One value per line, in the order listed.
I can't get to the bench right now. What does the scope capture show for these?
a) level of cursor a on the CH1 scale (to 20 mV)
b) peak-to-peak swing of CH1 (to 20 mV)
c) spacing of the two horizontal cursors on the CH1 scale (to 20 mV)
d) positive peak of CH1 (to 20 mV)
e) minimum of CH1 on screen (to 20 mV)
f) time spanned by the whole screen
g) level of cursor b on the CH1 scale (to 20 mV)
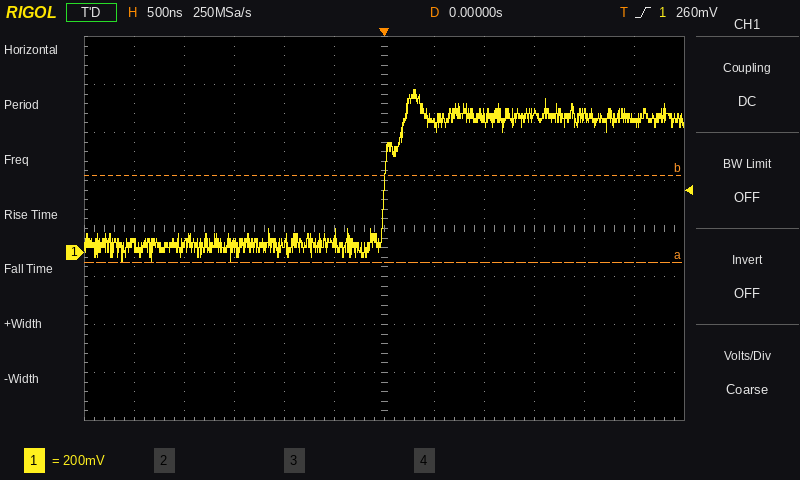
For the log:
-40 mV
720 mV
360 mV
680 mV
-40 mV
6 µs
320 mV
